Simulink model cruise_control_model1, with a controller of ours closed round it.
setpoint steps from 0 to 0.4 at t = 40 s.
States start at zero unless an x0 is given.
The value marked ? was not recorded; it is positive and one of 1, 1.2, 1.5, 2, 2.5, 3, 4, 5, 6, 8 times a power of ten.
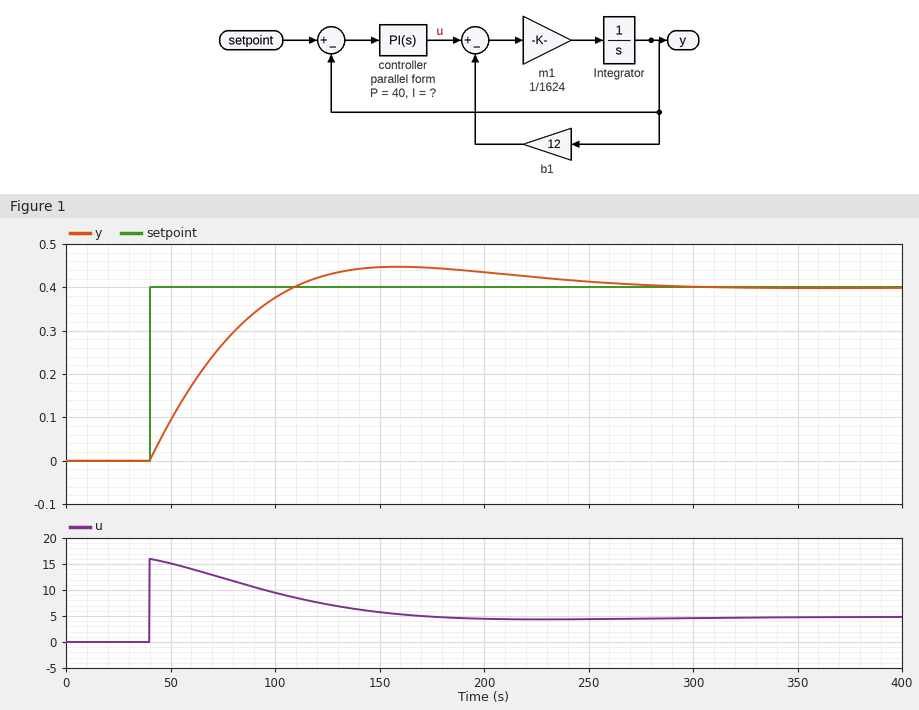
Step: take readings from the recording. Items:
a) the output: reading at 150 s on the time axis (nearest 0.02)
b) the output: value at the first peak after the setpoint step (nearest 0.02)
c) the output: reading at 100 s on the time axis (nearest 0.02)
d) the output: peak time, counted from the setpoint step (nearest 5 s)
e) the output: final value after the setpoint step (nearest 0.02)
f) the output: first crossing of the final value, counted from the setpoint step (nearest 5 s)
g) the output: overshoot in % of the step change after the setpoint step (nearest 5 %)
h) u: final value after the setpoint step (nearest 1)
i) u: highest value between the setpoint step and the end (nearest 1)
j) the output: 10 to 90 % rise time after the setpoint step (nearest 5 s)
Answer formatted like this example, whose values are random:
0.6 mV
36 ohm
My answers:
0.44
0.44
0.38
120 s
0.40
70 s
10 %
5
16
50 s
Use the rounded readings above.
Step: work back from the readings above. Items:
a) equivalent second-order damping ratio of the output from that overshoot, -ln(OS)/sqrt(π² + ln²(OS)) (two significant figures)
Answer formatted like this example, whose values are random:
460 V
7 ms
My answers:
0.59
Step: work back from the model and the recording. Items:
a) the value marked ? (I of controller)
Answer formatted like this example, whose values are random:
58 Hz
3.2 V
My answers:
0.8
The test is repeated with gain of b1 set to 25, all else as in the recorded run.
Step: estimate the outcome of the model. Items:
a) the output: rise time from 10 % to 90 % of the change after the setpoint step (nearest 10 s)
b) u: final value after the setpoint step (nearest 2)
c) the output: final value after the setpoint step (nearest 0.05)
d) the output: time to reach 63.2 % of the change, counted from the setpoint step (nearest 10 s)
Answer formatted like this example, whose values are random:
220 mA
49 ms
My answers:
70 s
10
0.40
40 s
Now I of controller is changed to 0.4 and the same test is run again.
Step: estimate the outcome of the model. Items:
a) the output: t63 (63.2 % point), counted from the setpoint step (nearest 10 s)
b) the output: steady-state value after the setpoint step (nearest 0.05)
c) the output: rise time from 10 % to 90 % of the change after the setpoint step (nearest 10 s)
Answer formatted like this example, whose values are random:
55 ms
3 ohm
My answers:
40 s
0.40
70 s
